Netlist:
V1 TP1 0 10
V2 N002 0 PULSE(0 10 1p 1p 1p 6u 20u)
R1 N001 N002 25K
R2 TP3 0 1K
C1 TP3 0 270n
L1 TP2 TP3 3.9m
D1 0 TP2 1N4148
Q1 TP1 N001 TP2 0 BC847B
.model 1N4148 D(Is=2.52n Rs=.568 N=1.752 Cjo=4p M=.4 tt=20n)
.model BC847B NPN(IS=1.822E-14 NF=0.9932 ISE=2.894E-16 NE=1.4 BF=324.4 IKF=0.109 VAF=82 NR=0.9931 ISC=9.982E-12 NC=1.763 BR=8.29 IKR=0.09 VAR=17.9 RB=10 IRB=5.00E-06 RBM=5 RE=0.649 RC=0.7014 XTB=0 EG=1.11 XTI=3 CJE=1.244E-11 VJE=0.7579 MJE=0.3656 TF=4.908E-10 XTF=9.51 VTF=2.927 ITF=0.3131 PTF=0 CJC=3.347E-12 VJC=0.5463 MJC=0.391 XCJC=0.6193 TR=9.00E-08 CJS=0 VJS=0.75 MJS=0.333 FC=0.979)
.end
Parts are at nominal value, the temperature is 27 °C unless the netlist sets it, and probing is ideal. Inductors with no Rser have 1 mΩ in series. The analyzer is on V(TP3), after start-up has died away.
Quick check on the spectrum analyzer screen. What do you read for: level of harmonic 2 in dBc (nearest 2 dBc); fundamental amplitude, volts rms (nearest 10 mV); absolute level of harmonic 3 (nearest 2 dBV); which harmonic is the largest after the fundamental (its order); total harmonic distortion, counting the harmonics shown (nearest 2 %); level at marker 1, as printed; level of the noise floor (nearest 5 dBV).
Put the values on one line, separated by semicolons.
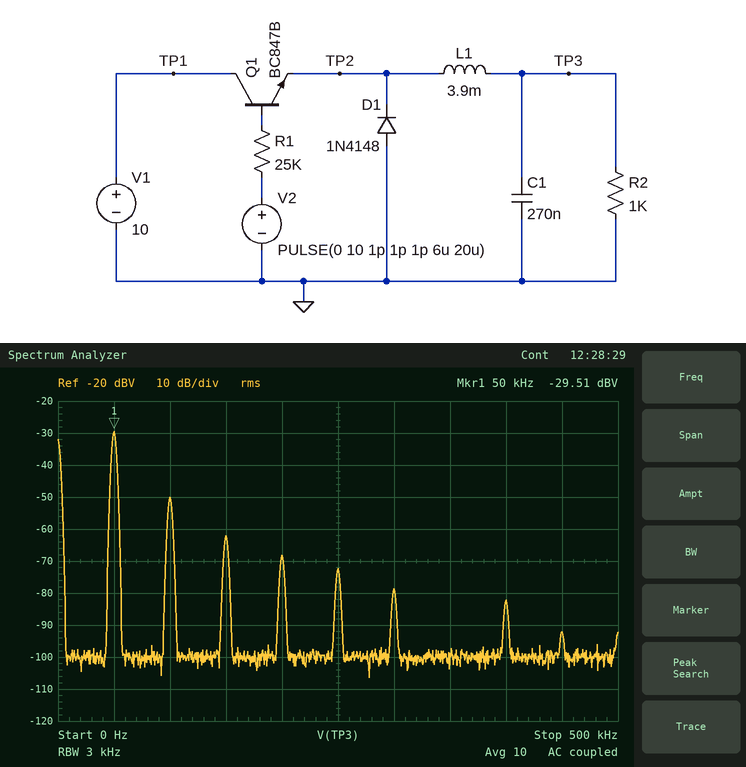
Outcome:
-20 dBc; 30 mV; -62 dBV; 2; 10 %; -29.51 dBV; -100 dBV
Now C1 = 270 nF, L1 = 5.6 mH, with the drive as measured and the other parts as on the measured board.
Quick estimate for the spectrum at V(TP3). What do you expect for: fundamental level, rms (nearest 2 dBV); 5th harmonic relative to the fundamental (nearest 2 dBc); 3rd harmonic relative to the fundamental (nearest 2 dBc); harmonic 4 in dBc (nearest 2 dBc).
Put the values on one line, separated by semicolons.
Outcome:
-32 dBV; -42 dBc; -36 dBc; -46 dBc
